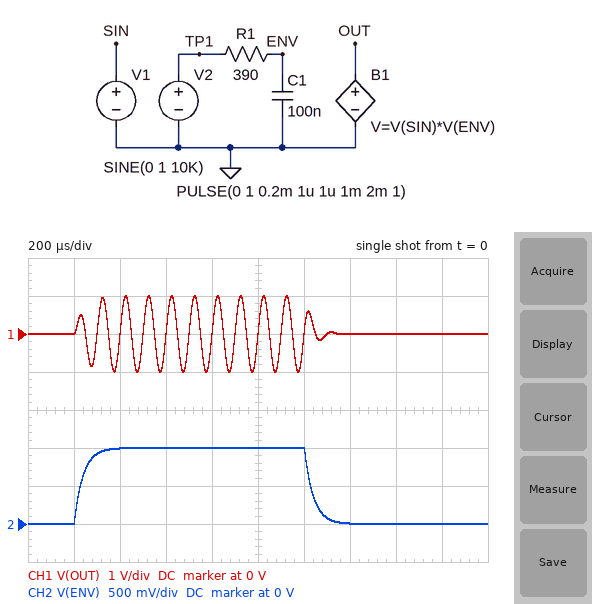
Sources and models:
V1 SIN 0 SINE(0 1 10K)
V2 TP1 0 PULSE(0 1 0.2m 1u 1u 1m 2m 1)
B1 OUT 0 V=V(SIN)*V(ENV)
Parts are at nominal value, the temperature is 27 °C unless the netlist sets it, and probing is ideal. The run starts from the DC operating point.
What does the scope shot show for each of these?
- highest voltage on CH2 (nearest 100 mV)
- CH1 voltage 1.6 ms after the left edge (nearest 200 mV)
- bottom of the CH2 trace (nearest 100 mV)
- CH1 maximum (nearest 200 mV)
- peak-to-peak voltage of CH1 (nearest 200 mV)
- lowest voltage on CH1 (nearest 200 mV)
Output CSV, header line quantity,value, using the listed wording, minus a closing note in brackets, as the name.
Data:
quantity,value
highest voltage on CH2,1.0 V
CH1 voltage 1.6 ms after the left edge,0 V
bottom of the CH2 trace,0 V
CH1 maximum,1.0 V
peak-to-peak voltage of CH1,2.0 V
lowest voltage on CH1,-1.0 V
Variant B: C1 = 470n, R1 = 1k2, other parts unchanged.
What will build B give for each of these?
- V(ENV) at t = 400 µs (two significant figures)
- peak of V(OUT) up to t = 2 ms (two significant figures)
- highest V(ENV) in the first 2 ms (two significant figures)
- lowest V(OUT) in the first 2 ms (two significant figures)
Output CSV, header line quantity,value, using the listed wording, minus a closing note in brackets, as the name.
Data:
quantity,value
V(ENV) at t = 400 µs,300 mV
peak of V(OUT) up to t = 2 ms,810 mV
highest V(ENV) in the first 2 ms,830 mV
lowest V(OUT) in the first 2 ms,-820 mV
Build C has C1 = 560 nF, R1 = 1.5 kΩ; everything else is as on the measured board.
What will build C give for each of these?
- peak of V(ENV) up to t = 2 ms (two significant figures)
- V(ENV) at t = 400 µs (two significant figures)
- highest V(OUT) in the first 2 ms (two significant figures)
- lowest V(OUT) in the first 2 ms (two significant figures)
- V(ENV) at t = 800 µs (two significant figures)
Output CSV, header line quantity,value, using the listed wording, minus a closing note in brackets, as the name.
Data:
quantity,value
peak of V(ENV) up to t = 2 ms,700 mV
V(ENV) at t = 400 µs,210 mV
highest V(OUT) in the first 2 ms,680 mV
lowest V(OUT) in the first 2 ms,-690 mV
V(ENV) at t = 800 µs,510 mV
